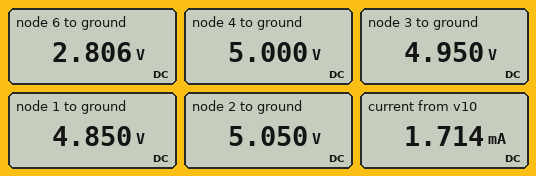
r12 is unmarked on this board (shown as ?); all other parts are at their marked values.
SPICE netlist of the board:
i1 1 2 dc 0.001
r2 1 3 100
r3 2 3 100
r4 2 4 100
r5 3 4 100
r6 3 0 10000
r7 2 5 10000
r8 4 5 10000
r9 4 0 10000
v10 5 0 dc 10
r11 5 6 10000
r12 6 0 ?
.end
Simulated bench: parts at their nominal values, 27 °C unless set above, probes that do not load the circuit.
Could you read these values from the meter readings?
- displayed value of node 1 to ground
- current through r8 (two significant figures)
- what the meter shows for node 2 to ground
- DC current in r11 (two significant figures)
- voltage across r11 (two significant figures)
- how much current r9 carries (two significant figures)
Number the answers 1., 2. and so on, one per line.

1. 4.850 V
2. 500 µA
3. 5.050 V
4. 720 µA
5. 7.2 V
6. 500 µA
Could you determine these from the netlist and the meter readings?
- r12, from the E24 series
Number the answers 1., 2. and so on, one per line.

1. 3.9 kΩ
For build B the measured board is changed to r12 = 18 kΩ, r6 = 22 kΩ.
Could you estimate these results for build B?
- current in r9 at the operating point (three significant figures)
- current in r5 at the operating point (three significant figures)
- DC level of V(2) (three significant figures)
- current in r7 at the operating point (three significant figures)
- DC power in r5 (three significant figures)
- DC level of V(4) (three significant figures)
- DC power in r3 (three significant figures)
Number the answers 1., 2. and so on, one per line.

1. 578 µA
2. 368 µA
3. 5.83 V
4. 417 µA
5. 13.6 µW
6. 5.78 V
7. 79.7 µW
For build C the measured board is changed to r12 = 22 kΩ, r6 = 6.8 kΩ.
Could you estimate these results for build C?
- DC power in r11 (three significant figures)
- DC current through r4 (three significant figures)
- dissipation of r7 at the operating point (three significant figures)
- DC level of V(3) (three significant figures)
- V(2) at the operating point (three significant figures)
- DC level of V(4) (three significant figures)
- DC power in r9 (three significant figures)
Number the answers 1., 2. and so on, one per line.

1. 977 µW
2. 481 µA
3. 2.99 mW
4. 4.42 V
5. 4.53 V
6. 4.48 V
7. 2.01 mW
